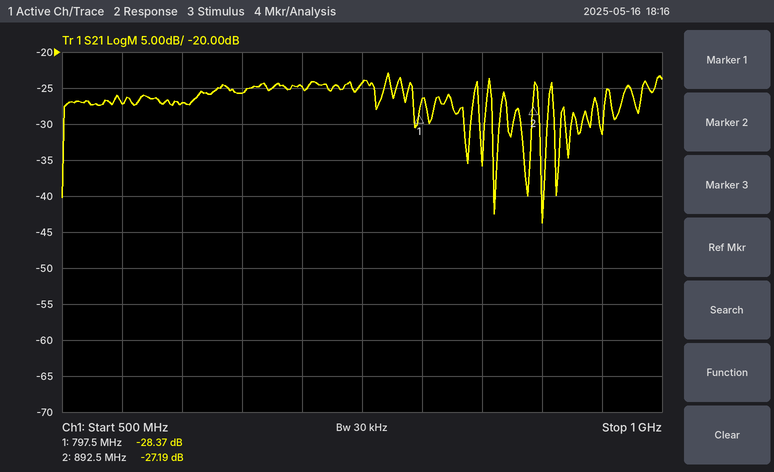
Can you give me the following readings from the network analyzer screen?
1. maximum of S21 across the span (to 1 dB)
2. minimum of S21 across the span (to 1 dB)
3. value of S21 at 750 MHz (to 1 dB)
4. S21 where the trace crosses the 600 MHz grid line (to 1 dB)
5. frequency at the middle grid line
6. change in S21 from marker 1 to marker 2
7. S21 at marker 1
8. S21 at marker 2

-23 dB
-44 dB
-24 dB
-27 dB
750 MHz
1.18 dB
-28.37 dB
-27.19 dB
